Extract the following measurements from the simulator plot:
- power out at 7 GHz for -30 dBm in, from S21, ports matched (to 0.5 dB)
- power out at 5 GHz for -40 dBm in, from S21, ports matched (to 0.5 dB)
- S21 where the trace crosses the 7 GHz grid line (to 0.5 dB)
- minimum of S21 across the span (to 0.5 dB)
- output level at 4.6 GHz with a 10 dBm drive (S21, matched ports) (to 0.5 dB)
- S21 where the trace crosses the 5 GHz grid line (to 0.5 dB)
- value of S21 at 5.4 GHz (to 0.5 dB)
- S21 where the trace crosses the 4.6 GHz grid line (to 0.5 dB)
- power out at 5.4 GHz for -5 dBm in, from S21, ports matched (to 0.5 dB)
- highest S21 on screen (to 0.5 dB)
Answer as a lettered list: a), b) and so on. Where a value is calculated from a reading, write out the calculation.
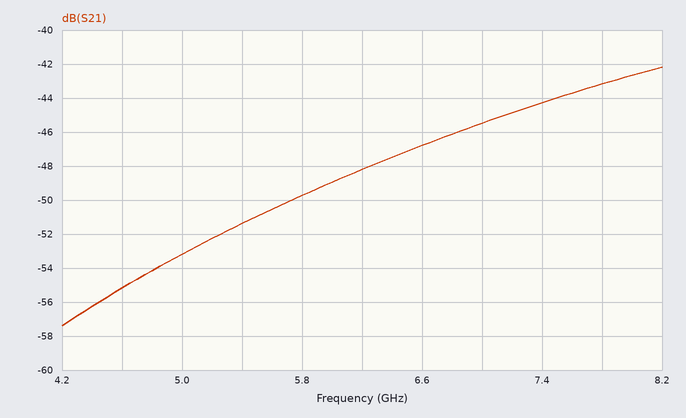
a) -30 dBm + (-45.5 dB) = -75.5 dBm
b) -40 dBm + (-53.0 dB) = -93.0 dBm
c) -45.5 dB
d) -57.5 dB
e) 10 dBm + (-55.0 dB) = -45.0 dBm
f) -53.0 dB
g) -51.5 dB
h) -55.0 dB
i) -5 dBm + (-51.5 dB) = -56.5 dBm
j) -42.0 dB
